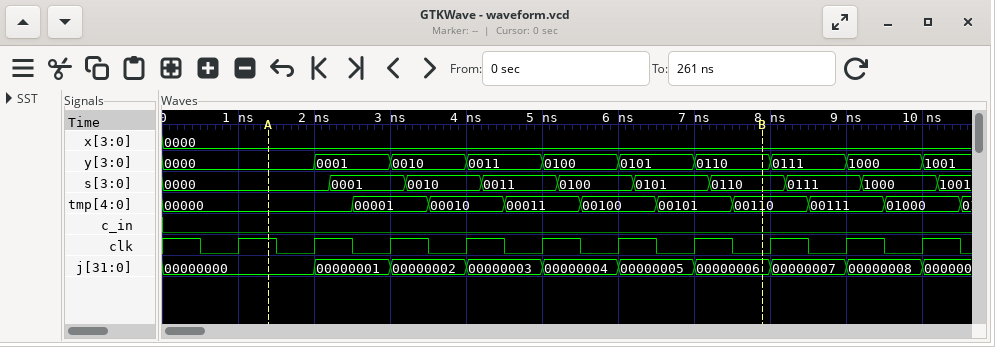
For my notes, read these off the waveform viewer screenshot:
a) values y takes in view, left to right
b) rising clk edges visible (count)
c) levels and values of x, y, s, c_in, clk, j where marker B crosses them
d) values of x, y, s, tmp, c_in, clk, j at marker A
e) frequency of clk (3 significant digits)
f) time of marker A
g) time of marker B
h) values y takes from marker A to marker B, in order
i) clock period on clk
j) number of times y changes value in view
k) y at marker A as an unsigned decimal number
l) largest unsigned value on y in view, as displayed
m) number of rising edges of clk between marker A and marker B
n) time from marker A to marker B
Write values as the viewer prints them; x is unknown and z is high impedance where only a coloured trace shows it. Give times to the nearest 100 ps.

0000, 0001, 0010, 0011, 0100, 0101, 0110, 0111, 1000, 1001
10
x=0000, y=0110, s=0110, c_in=0, clk=0, j=00000006
x=0000, y=0000, s=0000, tmp=00000, c_in=0, clk=1, j=00000000
1.00 GHz
1400 ps
7900 ps
0000, 0001, 0010, 0011, 0100, 0101, 0110
1000 ps
9
0
1001
6
6500 ps
